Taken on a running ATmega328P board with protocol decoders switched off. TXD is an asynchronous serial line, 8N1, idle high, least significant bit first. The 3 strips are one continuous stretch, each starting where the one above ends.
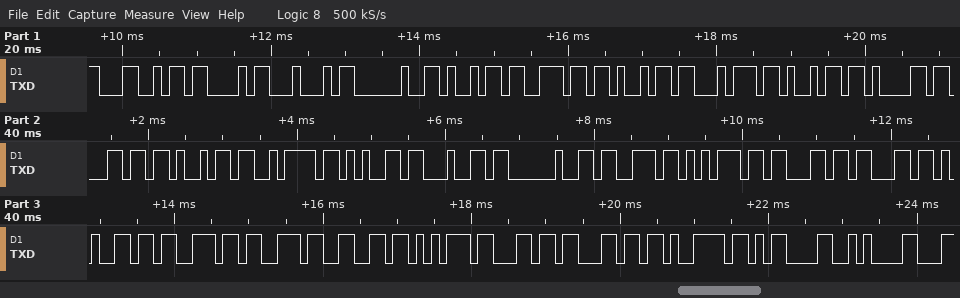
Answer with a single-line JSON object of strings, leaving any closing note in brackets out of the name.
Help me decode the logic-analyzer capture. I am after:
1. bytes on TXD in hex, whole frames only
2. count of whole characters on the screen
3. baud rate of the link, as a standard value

{"bytes on TXD in hex, whole frames only": "0x4C 0x43 0x44 0x20 0x69 0x6E 0x69 0x74 0x69 0x61 0x6C 0x69 0x7A 0x65 0x64 0x20 0x73 0x75 0x63 0x63 0x65 0x73 0x73 0x66 0x75 0x6C 0x6C 0x79 0x0D 0x0A", "count of whole characters on the screen": "30", "baud rate of the link, as a standard value": "9600 baud"}
